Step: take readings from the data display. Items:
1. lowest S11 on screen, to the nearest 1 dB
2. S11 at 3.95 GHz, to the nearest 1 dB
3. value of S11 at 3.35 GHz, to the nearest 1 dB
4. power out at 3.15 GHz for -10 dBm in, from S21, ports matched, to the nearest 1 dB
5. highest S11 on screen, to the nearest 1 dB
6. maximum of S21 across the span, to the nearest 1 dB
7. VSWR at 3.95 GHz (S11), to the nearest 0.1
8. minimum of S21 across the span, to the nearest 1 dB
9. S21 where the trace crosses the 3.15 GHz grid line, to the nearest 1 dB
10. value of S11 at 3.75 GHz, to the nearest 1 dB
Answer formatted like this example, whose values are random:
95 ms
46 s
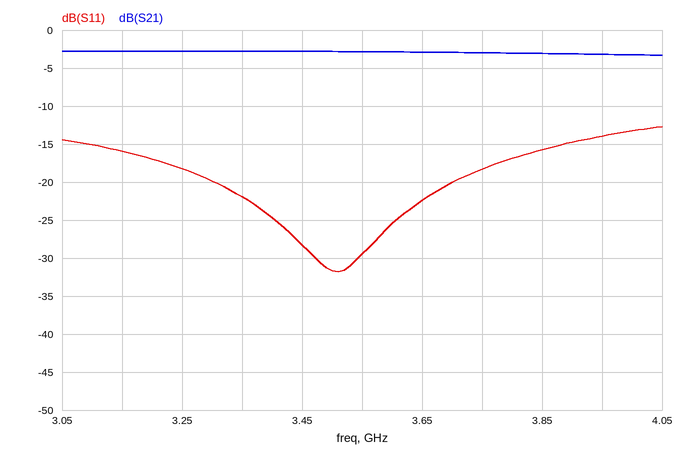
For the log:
-32 dB
-14 dB
-22 dB
-13 dBm
-13 dB
-3 dB
1.5
-3 dB
-3 dB
-18 dB
